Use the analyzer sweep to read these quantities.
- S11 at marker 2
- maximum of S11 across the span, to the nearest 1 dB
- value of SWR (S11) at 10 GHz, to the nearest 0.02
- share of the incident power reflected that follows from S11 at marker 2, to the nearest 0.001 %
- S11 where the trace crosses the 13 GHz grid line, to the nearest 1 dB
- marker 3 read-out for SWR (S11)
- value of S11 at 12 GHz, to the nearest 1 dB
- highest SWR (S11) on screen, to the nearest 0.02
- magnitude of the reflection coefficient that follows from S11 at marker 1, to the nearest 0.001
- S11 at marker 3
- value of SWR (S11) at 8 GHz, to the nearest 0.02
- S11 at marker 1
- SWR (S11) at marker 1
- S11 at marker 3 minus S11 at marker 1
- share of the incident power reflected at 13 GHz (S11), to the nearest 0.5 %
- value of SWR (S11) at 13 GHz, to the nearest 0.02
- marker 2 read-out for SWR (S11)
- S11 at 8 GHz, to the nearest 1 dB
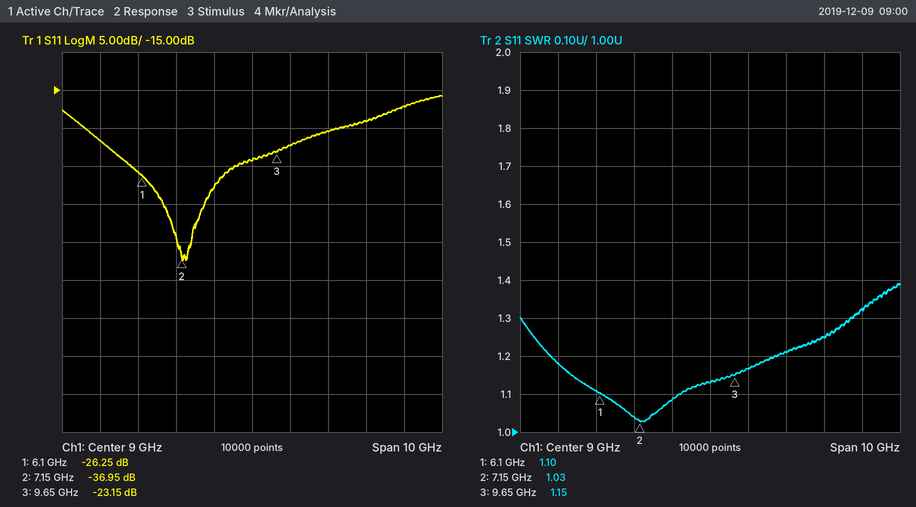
-36.95 dB
-16 dB
1.16
0.020 %
-17 dB
1.15
-19 dB
1.40
0.049
-23.15 dB
1.08
-26.25 dB
1.10
3.10 dB
2.0 %
1.32
1.03
-28 dB
